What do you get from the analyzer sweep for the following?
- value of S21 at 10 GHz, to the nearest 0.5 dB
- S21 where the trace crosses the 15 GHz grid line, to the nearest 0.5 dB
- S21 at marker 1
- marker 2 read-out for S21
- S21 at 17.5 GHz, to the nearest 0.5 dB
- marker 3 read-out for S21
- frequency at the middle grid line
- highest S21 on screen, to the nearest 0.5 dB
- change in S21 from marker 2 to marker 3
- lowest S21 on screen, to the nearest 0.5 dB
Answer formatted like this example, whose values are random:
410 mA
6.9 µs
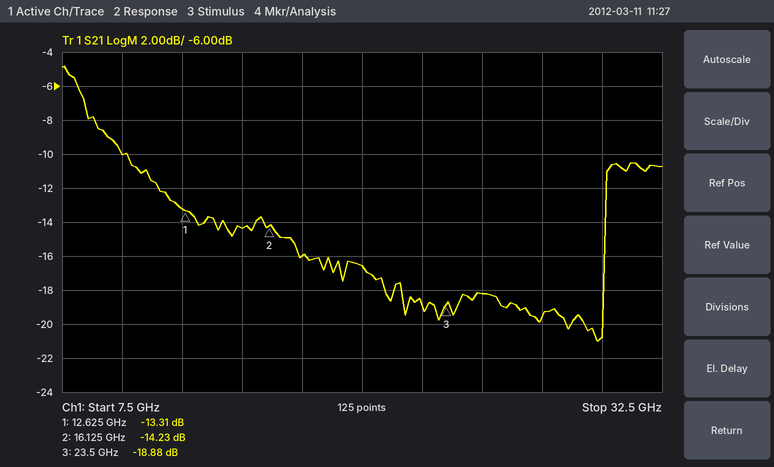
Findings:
-10.0 dB
-14.5 dB
-13.31 dB
-14.23 dB
-16.0 dB
-18.88 dB
20 GHz
-5.0 dB
-4.65 dB
-21.0 dB
